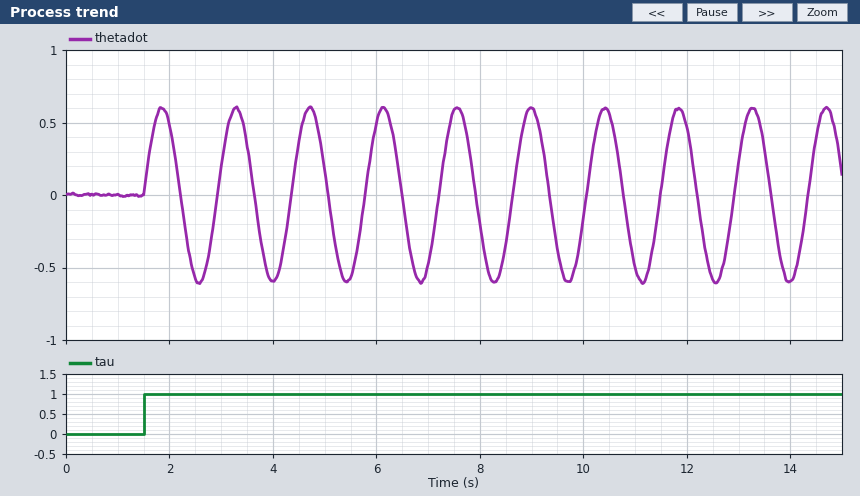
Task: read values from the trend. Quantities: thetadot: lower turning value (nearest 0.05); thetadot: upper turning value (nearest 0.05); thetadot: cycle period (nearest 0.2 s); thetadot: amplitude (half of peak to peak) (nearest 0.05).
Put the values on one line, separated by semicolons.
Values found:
-0.60; 0.60; 1.4 s; 0.60
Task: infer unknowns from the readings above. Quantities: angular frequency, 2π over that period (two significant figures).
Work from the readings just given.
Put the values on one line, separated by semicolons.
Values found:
4.5 rad/s
